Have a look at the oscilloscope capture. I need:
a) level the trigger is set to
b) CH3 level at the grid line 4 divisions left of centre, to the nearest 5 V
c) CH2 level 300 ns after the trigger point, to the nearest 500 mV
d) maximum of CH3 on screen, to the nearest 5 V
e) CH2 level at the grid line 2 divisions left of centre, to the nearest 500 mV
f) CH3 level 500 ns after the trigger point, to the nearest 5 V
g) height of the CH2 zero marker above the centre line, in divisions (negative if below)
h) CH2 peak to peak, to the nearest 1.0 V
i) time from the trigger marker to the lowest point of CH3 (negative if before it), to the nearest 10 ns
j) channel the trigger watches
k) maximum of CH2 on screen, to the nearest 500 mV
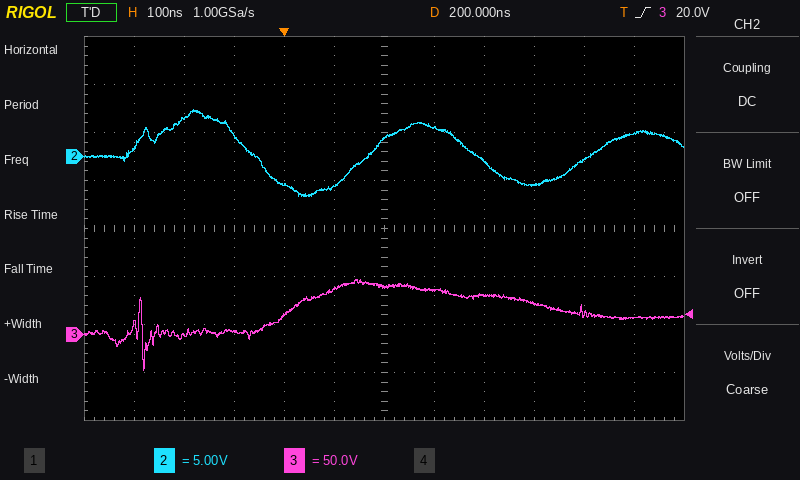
20.0 V
0 V
3.0 V
55 V
-3.0 V
30 V
+1.5 div
9.0 V
-280 ns
CH3
5.0 V
